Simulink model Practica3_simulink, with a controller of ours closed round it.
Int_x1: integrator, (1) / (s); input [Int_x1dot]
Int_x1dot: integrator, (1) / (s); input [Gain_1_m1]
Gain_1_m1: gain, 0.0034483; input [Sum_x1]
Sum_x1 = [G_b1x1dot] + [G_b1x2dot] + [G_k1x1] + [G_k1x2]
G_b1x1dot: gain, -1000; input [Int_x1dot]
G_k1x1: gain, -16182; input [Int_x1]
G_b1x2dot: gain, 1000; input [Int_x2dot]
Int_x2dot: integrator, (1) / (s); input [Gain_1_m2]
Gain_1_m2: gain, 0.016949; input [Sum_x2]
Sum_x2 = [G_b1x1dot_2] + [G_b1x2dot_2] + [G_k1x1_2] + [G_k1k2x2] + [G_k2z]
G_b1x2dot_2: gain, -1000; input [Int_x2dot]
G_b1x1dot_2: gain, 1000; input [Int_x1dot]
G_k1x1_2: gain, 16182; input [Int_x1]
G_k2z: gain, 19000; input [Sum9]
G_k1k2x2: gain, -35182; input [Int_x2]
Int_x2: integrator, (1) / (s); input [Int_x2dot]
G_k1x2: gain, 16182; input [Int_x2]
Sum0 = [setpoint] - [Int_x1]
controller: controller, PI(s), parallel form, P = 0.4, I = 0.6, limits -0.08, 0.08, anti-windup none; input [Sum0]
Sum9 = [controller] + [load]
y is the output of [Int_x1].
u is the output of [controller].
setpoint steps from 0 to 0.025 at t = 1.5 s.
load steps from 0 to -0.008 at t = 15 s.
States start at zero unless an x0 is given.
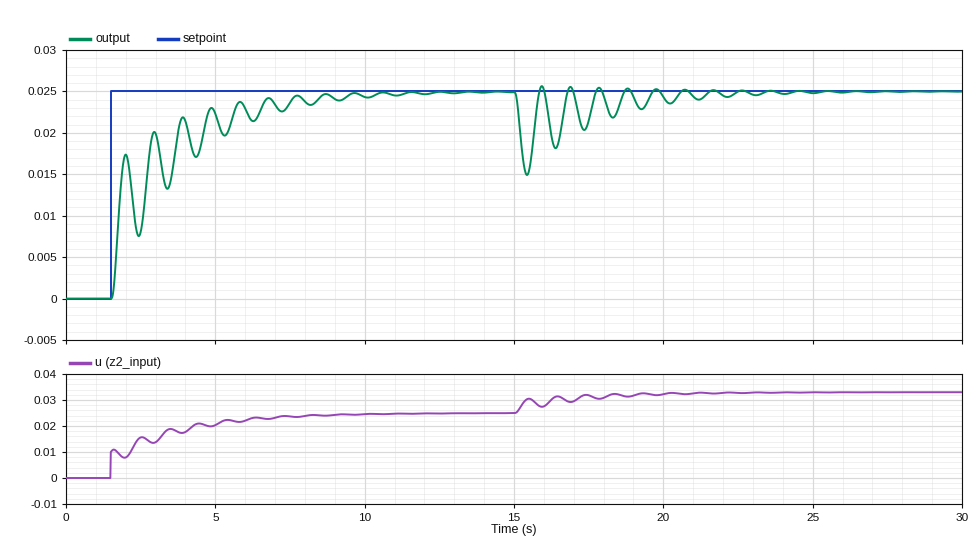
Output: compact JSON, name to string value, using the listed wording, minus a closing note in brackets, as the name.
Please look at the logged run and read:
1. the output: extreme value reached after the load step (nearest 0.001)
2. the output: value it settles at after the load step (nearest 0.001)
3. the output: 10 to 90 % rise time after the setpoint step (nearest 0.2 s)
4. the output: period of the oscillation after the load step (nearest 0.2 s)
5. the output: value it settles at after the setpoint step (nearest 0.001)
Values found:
{"the output: extreme value reached after the load step": "0.015", "the output: value it settles at after the load step": "0.025", "the output: 10 to 90 % rise time after the setpoint step": "3.2 s", "the output: period of the oscillation after the load step": "1.0 s", "the output: value it settles at after the setpoint step": "0.025"}
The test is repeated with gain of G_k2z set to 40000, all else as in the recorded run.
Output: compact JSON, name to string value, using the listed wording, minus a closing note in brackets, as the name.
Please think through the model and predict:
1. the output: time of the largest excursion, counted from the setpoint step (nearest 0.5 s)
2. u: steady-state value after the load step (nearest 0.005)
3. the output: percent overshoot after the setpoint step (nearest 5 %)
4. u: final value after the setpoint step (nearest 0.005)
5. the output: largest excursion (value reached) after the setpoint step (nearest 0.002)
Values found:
{"the output: time of the largest excursion, counted from the setpoint step": "2.0 s", "u: steady-state value after the load step": "0.020", "the output: percent overshoot after the setpoint step": "10 %", "u: final value after the setpoint step": "0.010", "the output: largest excursion (value reached) after the setpoint step": "0.028"}
